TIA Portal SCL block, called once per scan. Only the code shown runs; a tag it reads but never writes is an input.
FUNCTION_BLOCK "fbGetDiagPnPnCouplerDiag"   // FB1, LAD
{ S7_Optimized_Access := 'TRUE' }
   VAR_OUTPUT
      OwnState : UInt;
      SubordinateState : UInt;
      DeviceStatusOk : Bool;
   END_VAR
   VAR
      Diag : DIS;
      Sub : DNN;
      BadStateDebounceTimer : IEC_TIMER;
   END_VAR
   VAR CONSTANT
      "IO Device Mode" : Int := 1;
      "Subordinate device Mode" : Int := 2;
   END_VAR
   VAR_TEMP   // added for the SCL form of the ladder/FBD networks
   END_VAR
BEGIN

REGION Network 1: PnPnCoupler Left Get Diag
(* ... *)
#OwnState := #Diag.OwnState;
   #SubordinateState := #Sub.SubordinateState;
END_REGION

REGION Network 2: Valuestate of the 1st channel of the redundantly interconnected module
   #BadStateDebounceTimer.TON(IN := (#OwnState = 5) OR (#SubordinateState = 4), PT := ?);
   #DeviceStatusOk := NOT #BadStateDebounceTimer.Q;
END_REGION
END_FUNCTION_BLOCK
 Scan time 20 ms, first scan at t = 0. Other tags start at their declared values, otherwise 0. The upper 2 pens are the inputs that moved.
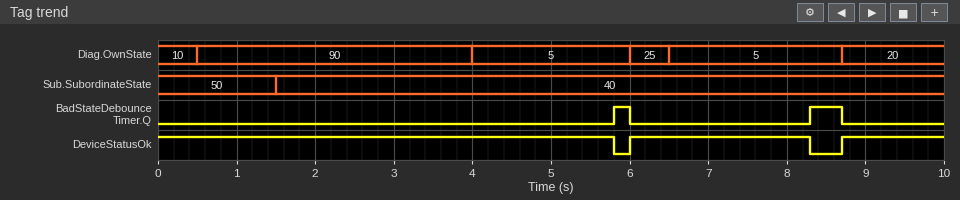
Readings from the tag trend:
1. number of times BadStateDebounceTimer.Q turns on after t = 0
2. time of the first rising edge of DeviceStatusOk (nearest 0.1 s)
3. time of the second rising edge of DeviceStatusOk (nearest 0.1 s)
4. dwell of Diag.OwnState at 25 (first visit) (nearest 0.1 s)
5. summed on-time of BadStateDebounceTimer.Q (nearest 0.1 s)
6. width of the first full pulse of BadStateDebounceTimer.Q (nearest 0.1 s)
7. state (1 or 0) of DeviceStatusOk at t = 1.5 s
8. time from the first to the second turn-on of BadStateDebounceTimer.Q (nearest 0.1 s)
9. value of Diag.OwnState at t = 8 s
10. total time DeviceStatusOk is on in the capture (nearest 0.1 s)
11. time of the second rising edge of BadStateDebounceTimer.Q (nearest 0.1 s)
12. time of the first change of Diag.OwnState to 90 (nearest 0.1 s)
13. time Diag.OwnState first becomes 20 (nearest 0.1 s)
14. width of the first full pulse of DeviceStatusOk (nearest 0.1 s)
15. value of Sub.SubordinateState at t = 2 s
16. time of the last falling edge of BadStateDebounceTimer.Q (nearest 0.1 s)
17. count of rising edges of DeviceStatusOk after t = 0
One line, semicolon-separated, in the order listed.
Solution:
2; 6.0 s; 8.7 s; 0.5 s; 0.6 s; 0.2 s; 1; 2.5 s; 5; 9.4 s; 8.3 s; 0.5 s; 8.7 s; 2.3 s; 40; 8.7 s; 2
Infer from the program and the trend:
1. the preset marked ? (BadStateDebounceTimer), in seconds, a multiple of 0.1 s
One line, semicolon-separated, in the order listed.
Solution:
1.8 s
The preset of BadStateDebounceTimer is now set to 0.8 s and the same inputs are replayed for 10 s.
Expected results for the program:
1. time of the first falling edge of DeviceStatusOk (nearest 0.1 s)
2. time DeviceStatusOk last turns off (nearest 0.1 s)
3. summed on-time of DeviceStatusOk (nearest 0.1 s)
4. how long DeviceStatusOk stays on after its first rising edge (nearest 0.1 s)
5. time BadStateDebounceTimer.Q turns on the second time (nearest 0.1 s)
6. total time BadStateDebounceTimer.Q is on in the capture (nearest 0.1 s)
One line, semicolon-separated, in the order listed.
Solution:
4.8 s; 7.3 s; 7.4 s; 1.3 s; 7.3 s; 2.6 s
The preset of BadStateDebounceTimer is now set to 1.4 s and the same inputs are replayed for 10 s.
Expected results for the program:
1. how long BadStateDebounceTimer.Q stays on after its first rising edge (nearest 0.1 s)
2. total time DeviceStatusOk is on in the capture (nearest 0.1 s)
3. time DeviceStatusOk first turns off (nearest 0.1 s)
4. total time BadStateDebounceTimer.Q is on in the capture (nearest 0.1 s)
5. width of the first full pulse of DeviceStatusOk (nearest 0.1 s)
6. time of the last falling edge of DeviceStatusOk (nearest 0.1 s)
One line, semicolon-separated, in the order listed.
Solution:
0.6 s; 8.6 s; 5.4 s; 1.4 s; 1.9 s; 7.9 s
